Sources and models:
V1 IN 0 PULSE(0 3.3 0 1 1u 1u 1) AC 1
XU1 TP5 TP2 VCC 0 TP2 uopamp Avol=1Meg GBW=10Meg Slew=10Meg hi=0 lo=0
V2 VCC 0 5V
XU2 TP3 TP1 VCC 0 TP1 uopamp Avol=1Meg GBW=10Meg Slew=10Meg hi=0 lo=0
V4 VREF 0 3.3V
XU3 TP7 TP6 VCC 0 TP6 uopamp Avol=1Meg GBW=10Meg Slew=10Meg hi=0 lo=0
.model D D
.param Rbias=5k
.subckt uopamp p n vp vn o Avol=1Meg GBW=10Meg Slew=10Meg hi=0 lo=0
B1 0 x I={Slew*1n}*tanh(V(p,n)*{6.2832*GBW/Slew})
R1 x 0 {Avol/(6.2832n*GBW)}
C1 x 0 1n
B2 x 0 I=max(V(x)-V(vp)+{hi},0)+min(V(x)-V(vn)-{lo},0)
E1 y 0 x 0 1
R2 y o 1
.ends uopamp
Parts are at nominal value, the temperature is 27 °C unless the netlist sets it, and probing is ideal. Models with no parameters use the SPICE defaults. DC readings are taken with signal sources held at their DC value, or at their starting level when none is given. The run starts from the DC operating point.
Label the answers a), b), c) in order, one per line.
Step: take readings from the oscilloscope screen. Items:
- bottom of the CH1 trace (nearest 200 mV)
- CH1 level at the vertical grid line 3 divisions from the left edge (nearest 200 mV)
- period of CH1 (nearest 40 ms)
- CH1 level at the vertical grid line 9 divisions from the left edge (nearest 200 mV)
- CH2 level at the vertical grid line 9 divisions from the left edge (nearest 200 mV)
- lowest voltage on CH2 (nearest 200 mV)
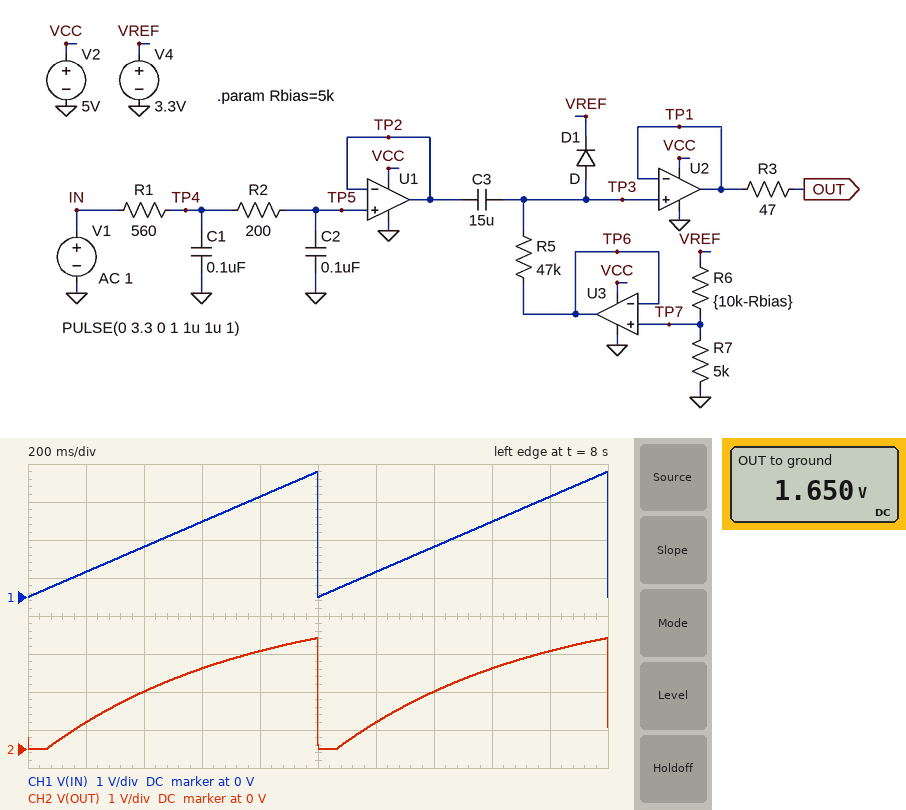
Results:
a) 0 V
b) 2.0 V
c) 1.00 s
d) 2.6 V
e) 2.6 V
f) 0 V
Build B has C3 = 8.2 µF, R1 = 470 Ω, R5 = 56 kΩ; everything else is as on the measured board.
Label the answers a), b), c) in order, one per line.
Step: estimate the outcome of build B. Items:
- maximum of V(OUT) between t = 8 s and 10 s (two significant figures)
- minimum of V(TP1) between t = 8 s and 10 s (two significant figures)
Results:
a) 2.7 V
b) -10 mV
